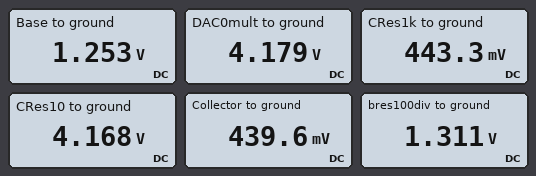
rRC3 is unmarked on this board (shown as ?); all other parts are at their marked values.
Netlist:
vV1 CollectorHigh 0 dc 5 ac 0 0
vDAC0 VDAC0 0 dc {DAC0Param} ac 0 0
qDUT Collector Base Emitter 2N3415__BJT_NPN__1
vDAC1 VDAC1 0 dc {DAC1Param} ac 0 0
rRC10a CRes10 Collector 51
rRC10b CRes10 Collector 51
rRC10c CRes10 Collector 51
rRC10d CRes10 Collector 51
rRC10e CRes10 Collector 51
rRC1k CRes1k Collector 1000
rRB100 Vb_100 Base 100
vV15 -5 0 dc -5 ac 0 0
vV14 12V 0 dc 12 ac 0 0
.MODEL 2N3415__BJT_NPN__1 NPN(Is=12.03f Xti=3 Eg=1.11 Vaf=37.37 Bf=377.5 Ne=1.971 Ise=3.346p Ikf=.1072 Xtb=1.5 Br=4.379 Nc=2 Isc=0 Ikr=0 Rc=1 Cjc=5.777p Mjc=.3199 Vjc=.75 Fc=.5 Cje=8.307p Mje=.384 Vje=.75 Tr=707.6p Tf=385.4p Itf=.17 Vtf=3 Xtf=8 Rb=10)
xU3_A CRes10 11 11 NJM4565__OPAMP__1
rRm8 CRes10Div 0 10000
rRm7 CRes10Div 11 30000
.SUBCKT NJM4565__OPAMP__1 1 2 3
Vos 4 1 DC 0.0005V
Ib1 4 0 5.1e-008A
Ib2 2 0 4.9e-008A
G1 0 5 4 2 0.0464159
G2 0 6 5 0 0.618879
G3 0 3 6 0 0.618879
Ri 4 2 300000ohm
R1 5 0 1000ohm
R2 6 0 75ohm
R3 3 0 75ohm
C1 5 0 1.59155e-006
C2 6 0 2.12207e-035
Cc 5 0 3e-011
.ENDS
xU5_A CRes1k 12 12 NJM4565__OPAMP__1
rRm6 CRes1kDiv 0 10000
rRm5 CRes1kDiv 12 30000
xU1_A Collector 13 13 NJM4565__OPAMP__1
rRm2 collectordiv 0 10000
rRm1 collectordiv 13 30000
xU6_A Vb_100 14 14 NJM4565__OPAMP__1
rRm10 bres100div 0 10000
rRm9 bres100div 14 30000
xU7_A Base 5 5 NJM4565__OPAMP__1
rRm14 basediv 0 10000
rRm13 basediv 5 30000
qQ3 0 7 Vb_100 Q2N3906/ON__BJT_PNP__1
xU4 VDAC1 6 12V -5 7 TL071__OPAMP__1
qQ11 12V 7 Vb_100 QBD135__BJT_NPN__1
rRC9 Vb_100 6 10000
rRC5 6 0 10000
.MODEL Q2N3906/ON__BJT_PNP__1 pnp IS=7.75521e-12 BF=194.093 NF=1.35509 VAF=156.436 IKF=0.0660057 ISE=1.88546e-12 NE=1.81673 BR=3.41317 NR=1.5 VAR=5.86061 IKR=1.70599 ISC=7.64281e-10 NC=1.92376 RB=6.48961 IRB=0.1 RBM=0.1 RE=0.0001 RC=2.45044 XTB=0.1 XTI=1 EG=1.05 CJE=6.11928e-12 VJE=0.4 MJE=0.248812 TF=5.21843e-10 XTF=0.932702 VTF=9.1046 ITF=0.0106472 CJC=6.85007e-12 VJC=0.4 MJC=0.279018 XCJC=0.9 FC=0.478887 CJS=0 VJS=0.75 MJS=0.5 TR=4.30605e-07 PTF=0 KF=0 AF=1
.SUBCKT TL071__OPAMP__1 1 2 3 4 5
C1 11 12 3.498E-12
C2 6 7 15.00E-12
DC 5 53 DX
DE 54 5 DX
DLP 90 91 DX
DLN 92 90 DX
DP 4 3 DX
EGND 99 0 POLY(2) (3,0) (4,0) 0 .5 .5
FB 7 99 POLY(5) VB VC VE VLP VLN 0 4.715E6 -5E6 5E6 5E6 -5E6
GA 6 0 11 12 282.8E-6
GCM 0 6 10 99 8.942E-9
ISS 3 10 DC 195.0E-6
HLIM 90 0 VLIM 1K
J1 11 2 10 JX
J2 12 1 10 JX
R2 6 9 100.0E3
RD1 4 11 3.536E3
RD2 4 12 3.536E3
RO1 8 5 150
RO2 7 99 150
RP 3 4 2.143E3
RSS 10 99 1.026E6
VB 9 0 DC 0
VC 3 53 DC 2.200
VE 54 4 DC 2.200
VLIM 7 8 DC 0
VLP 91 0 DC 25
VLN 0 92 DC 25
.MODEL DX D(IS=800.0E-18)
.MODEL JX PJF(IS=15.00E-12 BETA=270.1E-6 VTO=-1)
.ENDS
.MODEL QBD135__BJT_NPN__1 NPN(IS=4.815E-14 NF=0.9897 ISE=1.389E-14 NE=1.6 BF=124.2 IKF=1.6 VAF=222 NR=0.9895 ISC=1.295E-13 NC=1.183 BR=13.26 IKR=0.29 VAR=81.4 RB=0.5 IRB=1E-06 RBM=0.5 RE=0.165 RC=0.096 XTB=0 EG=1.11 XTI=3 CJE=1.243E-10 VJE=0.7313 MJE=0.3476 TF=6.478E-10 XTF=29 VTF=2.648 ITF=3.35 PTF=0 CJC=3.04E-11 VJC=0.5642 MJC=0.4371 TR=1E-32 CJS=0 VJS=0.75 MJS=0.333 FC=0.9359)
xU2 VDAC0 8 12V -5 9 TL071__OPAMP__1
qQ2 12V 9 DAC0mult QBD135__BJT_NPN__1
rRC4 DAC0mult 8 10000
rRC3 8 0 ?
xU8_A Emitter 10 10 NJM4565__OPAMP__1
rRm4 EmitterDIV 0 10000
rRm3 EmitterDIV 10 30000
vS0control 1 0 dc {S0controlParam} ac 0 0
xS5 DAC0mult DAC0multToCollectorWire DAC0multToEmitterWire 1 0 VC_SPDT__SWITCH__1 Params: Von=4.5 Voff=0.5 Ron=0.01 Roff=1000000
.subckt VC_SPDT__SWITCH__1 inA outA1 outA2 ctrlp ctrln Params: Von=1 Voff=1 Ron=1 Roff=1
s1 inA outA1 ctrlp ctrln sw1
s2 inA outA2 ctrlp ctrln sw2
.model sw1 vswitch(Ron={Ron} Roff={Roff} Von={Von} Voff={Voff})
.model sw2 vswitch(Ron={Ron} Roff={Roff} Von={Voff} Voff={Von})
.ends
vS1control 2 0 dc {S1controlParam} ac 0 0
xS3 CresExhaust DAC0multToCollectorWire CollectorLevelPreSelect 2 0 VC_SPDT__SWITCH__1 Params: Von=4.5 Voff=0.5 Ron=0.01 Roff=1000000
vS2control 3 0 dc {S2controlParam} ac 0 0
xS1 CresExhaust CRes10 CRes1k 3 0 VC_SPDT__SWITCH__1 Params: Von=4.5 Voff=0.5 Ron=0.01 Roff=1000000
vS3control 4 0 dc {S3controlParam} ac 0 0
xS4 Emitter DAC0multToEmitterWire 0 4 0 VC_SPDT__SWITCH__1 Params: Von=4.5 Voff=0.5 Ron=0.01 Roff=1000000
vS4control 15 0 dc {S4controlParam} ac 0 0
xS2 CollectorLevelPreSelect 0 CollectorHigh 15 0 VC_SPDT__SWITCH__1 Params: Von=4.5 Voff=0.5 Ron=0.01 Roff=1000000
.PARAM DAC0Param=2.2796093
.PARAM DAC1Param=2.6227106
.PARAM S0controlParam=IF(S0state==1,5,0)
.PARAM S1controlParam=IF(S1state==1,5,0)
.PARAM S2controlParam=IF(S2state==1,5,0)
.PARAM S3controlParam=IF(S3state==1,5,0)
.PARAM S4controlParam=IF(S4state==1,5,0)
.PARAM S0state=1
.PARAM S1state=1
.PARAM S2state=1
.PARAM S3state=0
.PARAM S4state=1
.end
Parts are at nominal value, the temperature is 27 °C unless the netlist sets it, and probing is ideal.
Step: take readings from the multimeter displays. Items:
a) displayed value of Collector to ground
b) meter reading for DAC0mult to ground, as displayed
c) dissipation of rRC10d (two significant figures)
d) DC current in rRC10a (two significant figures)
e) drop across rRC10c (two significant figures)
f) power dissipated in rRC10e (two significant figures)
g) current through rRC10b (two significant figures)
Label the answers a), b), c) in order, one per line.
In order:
a) 439.6 mV
b) 4.179 V
c) 270 mW
d) 73 mA
e) 3.7 V
f) 270 mW
g) 73 mA
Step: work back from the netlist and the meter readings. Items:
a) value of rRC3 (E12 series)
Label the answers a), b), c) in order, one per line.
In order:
a) 12 kΩ
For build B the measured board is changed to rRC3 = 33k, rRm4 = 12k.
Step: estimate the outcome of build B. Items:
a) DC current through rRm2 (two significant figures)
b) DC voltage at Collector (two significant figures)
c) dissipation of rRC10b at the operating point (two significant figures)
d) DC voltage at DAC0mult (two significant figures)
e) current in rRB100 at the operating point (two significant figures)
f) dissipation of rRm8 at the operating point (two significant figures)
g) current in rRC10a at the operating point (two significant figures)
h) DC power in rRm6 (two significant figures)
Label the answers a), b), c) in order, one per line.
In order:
a) 8.0 µA
b) 320 mV
c) 140 mW
d) 3.0 V
e) 40 mA
f) 55 µW
g) 52 mA
h) 650 nW
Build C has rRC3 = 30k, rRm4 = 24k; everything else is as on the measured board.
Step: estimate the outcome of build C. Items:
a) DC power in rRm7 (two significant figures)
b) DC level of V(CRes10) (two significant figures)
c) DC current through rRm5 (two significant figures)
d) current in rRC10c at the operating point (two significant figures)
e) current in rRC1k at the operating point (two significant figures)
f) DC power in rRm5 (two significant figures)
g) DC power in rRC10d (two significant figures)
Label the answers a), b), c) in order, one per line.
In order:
a) 170 µW
b) 3.0 V
c) 8.2 µA
d) 53 mA
e) 2.7 µA
f) 2.0 µW
g) 140 mW
